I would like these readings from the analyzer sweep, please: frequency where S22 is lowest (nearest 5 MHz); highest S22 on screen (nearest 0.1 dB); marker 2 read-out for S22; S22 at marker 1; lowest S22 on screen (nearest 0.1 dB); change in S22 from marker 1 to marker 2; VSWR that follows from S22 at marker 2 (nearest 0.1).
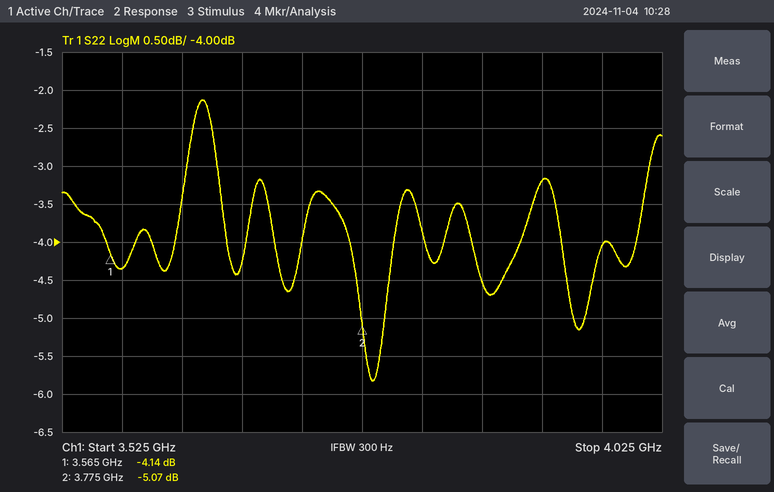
3.785 GHz
-2.1 dB
-5.07 dB
-4.14 dB
-5.8 dB
-0.93 dB
3.5
